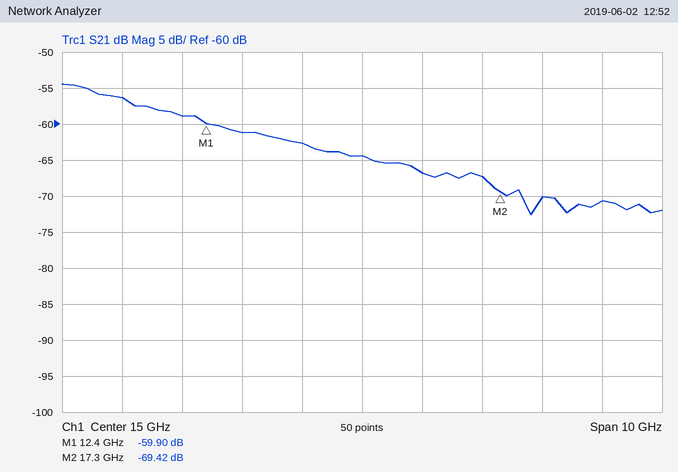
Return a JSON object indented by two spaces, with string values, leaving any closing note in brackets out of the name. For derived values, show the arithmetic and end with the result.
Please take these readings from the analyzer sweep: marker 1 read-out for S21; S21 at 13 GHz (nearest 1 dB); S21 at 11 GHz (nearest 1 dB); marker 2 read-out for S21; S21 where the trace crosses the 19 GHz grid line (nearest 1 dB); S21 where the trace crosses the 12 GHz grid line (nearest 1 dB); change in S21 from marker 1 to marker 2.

{
  "marker 1 read-out for S21": "-59.90 dB",
  "S21 at 13 GHz": "-61 dB",
  "S21 at 11 GHz": "-56 dB",
  "marker 2 read-out for S21": "-69.42 dB",
  "S21 where the trace crosses the 19 GHz grid line": "-71 dB",
  "S21 where the trace crosses the 12 GHz grid line": "-59 dB",
  "change in S21 from marker 1 to marker 2": "-69.42 − (-59.9) = -9.52 dB"
}
